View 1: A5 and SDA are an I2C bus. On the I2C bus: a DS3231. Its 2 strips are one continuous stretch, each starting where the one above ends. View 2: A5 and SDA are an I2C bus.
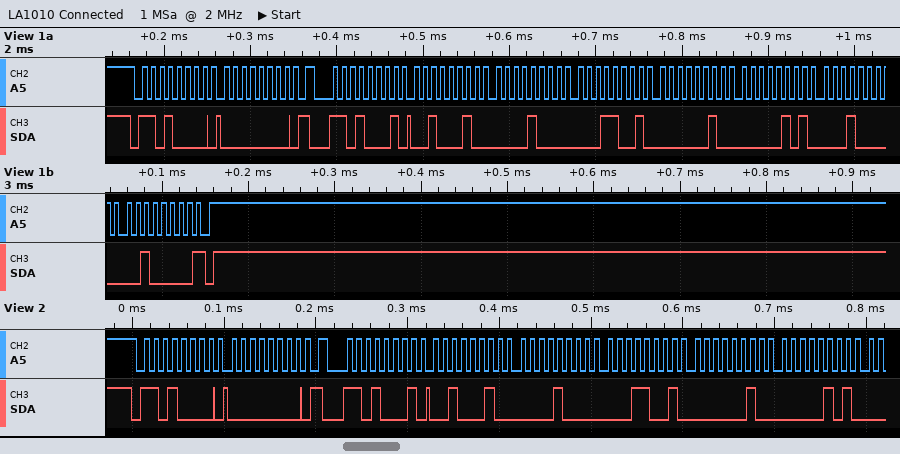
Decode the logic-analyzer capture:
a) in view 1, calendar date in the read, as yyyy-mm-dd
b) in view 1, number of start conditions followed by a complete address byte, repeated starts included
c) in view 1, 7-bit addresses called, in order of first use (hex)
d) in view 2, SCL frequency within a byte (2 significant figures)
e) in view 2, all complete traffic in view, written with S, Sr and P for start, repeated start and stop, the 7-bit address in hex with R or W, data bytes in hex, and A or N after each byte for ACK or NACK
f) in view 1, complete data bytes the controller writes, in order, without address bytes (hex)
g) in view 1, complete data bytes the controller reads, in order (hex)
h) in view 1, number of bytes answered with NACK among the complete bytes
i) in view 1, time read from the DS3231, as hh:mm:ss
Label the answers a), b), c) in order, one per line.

a) 2020-10-05
b) 2
c) 0x68
d) 100 kHz
e) S 68W A 00 A Sr 68R A 22 A 08 A 19 A 02 A 05 A
f) 00
g) 22 08 19 02 05 10 20
h) 1
i) 19:08:22
